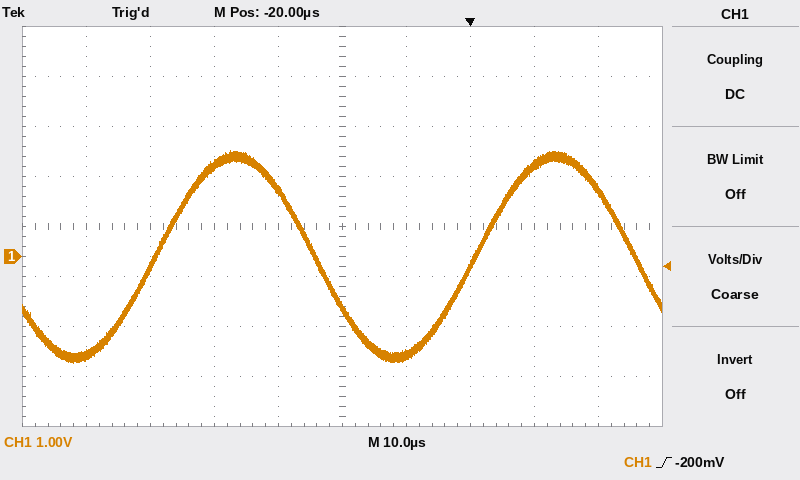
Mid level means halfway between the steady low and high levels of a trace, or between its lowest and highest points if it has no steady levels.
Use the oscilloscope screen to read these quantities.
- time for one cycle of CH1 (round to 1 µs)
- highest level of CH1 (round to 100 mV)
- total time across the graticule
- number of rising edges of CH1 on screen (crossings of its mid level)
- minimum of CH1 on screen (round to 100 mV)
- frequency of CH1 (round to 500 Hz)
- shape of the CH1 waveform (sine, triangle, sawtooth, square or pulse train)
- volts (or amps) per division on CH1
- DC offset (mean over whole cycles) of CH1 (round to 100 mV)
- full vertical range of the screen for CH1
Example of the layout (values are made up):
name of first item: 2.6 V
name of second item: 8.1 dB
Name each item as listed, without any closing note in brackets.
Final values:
time for one cycle of CH1: 50 µs
highest level of CH1: 2.1 V
total time across the graticule: 100 µs
number of rising edges of CH1 on screen: 2
minimum of CH1 on screen: -2.1 V
frequency of CH1: 20.0 kHz
shape of the CH1 waveform: sine
volts (or amps) per division on CH1: 1 V
DC offset (mean over whole cycles) of CH1: 0.0 V
full vertical range of the screen for CH1: 8 V
